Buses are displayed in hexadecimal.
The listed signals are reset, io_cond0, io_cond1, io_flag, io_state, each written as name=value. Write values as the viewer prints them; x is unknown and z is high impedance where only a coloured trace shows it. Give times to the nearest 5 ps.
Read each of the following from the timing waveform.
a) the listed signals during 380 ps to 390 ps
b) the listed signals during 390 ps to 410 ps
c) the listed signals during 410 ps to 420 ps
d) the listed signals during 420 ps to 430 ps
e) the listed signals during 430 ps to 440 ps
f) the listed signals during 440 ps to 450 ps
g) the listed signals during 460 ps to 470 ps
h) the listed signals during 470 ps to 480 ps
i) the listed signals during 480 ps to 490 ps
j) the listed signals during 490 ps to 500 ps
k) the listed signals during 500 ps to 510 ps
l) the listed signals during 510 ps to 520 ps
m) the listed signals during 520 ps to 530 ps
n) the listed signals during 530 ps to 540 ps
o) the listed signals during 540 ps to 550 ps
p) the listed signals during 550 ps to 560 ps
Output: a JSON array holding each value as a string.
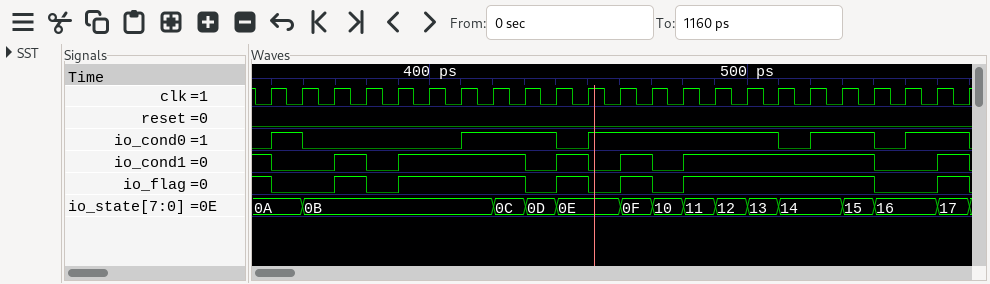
["reset=0, io_cond0=0, io_cond1=0, io_flag=0, io_state=0B", "reset=0, io_cond0=0, io_cond1=1, io_flag=1, io_state=0B", "reset=0, io_cond0=1, io_cond1=1, io_flag=1, io_state=0B", "reset=0, io_cond0=1, io_cond1=1, io_flag=1, io_state=0C", "reset=0, io_cond0=1, io_cond1=0, io_flag=0, io_state=0D", "reset=0, io_cond0=0, io_cond1=1, io_flag=1, io_state=0E", "reset=0, io_cond0=1, io_cond1=1, io_flag=1, io_state=0F", "reset=0, io_cond0=1, io_cond1=0, io_flag=0, io_state=10", "reset=0, io_cond0=1, io_cond1=1, io_flag=1, io_state=11", "reset=0, io_cond0=1, io_cond1=1, io_flag=1, io_state=12", "reset=0, io_cond0=1, io_cond1=1, io_flag=1, io_state=13", "reset=0, io_cond0=0, io_cond1=1, io_flag=1, io_state=14", "reset=0, io_cond0=1, io_cond1=1, io_flag=1, io_state=14", "reset=0, io_cond0=1, io_cond1=1, io_flag=1, io_state=15", "reset=0, io_cond0=0, io_cond1=0, io_flag=0, io_state=16", "reset=0, io_cond0=1, io_cond1=0, io_flag=0, io_state=16"]
